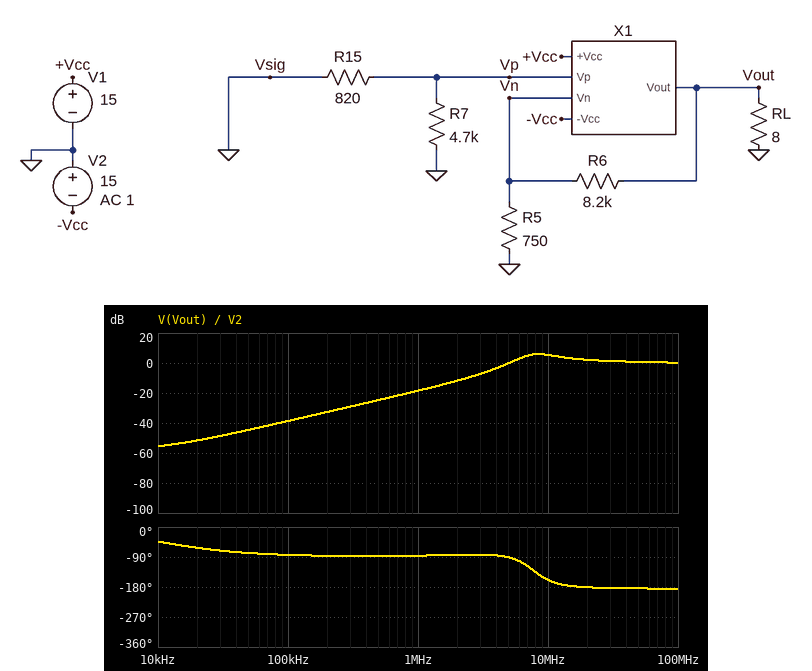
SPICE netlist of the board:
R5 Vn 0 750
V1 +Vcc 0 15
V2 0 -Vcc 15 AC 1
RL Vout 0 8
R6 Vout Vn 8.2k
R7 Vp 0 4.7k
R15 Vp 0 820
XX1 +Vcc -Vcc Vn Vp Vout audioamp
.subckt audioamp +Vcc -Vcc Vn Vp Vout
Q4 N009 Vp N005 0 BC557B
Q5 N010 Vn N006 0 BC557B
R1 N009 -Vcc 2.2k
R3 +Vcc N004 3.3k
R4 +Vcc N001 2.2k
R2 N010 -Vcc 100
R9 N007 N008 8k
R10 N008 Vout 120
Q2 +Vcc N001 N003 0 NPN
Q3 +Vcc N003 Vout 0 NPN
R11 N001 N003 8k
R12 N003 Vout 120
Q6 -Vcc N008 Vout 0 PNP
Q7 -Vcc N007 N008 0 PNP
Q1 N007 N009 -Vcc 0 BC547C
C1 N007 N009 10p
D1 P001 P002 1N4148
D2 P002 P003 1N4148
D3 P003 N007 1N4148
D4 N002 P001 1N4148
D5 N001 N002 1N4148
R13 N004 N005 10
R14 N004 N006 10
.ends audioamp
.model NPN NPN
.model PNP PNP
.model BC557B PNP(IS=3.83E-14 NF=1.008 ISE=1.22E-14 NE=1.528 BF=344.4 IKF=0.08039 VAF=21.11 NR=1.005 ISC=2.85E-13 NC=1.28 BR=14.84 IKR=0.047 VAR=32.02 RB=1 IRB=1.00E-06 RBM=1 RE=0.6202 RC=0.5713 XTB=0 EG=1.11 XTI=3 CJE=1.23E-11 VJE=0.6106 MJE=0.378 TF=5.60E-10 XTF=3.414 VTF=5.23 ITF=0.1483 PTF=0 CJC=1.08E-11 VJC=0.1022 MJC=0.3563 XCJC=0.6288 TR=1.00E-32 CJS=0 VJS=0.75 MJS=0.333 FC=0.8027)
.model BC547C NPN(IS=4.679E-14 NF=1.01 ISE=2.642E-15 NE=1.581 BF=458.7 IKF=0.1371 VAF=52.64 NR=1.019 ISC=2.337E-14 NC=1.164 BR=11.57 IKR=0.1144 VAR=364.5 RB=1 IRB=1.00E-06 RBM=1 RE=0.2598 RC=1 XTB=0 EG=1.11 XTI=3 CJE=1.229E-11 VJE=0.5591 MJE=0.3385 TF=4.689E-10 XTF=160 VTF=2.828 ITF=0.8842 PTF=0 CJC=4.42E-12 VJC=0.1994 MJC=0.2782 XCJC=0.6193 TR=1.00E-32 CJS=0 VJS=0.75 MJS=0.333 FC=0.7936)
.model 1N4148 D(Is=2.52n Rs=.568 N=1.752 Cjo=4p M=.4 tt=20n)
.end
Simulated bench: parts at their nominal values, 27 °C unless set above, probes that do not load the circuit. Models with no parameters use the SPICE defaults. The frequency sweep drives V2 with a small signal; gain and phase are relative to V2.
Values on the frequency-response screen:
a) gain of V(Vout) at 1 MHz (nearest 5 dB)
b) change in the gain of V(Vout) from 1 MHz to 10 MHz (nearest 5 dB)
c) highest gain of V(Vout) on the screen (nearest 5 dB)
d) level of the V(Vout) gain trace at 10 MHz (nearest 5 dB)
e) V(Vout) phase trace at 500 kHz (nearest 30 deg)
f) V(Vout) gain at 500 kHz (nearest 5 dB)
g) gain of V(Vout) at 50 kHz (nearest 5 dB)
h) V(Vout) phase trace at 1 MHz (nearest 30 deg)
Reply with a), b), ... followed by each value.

a) -20 dB
b) 25 dB
c) 5 dB
d) 5 dB
e) -90 deg
f) -25 dB
g) -45 dB
h) -90 deg
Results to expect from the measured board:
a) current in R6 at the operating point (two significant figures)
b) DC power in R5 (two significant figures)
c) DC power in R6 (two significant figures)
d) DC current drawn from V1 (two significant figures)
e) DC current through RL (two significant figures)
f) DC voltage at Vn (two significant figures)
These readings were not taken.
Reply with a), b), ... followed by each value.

a) 150 µA
b) 15 µW
c) 180 µW
d) 21 mA
e) 170 mA
f) -110 mV
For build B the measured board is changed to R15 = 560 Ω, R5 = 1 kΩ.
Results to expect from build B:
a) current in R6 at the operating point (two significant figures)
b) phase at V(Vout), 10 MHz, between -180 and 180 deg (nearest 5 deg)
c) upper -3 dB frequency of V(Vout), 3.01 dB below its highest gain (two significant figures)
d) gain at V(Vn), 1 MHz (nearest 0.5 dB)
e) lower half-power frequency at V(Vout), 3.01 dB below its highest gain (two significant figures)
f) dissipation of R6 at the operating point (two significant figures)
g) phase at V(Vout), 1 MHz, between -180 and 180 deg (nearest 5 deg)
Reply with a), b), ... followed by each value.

a) 110 µA
b) -120 deg
c) 19 MHz
d) -36.0 dB
e) 7.8 MHz
f) 110 µW
g) -75 deg
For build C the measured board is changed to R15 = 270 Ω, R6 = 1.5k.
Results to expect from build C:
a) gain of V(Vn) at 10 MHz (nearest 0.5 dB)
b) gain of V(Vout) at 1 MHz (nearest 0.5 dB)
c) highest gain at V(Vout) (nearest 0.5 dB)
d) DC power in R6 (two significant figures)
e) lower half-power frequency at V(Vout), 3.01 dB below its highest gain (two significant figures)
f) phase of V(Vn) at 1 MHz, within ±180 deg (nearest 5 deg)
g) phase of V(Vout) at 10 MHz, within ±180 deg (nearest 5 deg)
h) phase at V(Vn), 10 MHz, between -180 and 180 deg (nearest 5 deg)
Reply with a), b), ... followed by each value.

a) -16.0 dB
b) -34.0 dB
c) 10.5 dB
d) 34 µW
e) 19 MHz
f) -90 deg
g) -55 deg
h) -80 deg
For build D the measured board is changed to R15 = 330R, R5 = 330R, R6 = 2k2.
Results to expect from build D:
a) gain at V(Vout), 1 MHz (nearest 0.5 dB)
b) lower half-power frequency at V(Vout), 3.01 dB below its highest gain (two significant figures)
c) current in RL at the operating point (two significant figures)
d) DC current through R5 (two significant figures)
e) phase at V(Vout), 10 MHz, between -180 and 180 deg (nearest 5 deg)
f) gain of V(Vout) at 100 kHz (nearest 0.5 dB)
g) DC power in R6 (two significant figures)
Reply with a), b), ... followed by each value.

a) -22.5 dB
b) 11 MHz
c) 100 mA
d) 320 µA
e) -105 deg
f) -42.5 dB
g) 240 µW
